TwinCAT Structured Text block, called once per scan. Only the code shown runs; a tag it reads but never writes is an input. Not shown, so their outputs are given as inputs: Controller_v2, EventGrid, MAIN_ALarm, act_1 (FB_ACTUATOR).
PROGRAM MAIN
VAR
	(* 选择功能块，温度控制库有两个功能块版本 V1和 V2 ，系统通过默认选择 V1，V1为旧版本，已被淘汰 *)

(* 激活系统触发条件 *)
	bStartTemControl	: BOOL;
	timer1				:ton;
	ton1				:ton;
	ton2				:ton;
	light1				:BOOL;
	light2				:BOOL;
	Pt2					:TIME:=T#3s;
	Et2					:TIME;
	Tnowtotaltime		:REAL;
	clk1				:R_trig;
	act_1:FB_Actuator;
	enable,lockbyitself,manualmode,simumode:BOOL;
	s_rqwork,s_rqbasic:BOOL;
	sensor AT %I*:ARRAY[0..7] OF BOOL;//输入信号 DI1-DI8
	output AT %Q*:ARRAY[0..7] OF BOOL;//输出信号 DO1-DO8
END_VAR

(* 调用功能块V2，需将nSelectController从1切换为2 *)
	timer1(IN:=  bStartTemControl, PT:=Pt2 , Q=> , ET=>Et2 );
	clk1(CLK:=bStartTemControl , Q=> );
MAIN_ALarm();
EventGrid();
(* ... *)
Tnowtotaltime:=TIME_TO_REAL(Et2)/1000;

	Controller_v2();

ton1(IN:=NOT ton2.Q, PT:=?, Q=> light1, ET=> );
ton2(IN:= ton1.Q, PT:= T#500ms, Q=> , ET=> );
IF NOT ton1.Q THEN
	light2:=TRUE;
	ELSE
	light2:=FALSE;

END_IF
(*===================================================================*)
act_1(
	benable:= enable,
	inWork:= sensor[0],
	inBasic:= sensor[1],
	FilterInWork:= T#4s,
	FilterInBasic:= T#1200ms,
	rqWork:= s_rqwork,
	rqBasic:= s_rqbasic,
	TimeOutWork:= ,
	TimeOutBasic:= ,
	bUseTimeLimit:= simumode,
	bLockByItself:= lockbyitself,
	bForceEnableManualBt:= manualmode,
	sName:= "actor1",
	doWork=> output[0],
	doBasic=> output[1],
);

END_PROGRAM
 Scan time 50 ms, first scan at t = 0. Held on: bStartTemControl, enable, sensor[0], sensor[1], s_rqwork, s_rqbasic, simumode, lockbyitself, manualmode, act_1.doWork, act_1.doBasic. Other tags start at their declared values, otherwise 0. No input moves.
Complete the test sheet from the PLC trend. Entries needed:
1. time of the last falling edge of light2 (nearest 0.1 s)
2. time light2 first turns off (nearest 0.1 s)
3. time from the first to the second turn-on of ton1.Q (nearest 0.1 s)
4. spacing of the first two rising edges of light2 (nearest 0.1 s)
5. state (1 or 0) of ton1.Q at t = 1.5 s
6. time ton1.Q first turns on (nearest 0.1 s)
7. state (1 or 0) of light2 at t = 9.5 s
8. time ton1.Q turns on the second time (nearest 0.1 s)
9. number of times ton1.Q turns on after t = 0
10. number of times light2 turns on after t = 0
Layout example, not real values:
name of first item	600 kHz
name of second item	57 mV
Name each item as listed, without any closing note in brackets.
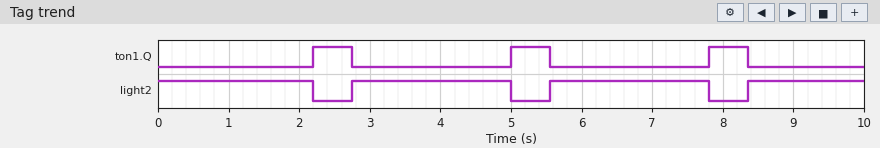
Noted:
time of the last falling edge of light2	7.8 s
time light2 first turns off	2.2 s
time from the first to the second turn-on of ton1.Q	2.8 s
spacing of the first two rising edges of light2	2.8 s
state (1 or 0) of ton1.Q at t = 1.5 s	0
time ton1.Q first turns on	2.2 s
state (1 or 0) of light2 at t = 9.5 s	1
time ton1.Q turns on the second time	5.0 s
number of times ton1.Q turns on after t = 0	3
number of times light2 turns on after t = 0	3
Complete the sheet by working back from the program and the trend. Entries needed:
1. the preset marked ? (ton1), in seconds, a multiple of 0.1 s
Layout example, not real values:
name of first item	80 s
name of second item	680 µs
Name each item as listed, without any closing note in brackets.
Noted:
the preset marked ? (ton1), in seconds, a multiple of 0.1 s	2.2 s
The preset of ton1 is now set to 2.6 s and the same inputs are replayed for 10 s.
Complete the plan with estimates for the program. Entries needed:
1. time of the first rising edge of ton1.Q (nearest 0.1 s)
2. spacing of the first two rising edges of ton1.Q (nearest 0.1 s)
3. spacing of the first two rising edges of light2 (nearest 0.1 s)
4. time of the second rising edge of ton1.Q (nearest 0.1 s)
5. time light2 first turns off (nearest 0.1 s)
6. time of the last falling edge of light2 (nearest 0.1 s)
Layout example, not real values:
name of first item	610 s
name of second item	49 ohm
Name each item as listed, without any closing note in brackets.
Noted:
time of the first rising edge of ton1.Q	2.6 s
spacing of the first two rising edges of ton1.Q	3.2 s
spacing of the first two rising edges of light2	3.2 s
time of the second rising edge of ton1.Q	5.8 s
time light2 first turns off	2.6 s
time of the last falling edge of light2	9.0 s
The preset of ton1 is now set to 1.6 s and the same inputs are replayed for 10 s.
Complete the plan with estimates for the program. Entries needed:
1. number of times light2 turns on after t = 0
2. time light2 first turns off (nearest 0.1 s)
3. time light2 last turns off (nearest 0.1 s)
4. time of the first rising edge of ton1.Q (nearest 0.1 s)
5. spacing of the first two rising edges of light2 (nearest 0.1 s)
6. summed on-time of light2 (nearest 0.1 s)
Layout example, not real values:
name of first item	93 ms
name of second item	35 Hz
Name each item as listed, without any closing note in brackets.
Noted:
number of times light2 turns on after t = 0	4
time light2 first turns off	1.6 s
time light2 last turns off	8.2 s
time of the first rising edge of ton1.Q	1.6 s
spacing of the first two rising edges of light2	2.2 s
summed on-time of light2	7.8 s
